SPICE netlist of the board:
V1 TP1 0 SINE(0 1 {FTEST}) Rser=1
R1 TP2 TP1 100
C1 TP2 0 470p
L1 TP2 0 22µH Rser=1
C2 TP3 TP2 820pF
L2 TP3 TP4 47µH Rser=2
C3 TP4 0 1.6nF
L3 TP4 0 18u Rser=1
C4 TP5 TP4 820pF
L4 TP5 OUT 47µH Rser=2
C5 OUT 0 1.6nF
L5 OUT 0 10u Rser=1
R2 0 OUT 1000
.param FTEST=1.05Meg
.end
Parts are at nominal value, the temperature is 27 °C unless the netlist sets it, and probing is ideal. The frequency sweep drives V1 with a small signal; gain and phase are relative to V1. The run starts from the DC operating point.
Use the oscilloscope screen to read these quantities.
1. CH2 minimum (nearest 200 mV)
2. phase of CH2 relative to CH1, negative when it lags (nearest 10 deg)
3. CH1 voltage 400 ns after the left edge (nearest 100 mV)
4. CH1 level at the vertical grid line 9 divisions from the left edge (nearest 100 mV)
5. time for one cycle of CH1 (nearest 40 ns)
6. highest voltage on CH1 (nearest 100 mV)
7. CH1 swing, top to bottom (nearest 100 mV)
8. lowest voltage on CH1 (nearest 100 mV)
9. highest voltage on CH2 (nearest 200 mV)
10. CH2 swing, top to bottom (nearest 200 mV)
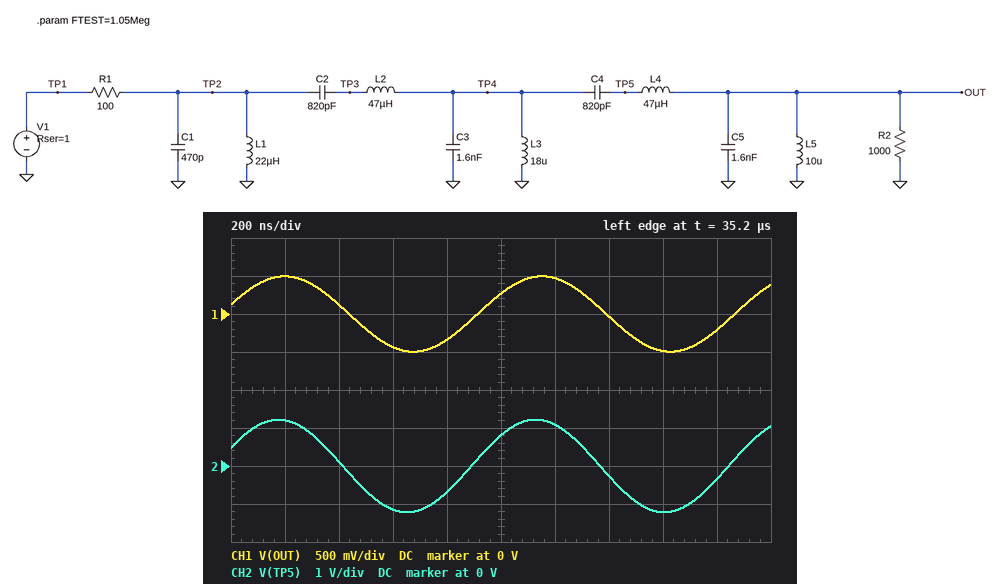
-1.2 V
10 deg
100 mV
-200 mV
960 ns
500 mV
1.0 V
-500 mV
1.2 V
2.4 V
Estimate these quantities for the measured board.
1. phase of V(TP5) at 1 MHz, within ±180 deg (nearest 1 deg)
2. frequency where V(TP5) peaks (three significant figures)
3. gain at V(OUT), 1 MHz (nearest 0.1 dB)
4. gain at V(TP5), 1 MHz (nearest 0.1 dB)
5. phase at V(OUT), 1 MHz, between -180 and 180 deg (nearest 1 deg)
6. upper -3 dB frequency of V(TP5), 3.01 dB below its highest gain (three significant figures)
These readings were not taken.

32 deg
713 kHz
-7.8 dB
1.0 dB
25 deg
768 kHz
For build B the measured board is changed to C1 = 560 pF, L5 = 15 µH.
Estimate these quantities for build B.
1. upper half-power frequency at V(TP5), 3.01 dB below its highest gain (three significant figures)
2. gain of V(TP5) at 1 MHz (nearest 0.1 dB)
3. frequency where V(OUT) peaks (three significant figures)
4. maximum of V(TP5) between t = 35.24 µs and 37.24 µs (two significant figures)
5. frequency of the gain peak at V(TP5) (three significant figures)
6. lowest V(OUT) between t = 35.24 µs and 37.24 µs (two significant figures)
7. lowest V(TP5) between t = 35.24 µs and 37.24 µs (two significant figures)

1.52 MHz
0.2 dB
1.11 MHz
1.1 V
1.47 MHz
-1.2 V
-1.1 V
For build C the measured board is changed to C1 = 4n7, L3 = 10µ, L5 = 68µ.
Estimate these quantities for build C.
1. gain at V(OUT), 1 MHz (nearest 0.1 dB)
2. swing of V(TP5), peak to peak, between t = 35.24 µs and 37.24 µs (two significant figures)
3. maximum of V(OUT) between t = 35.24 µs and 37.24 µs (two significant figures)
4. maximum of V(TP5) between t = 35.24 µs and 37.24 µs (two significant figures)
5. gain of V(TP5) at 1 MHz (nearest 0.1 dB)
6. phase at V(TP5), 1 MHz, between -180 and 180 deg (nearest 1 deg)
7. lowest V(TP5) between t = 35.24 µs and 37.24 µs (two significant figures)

0.5 dB
1.4 V
430 mV
690 mV
2.9 dB
-14 deg
-690 mV
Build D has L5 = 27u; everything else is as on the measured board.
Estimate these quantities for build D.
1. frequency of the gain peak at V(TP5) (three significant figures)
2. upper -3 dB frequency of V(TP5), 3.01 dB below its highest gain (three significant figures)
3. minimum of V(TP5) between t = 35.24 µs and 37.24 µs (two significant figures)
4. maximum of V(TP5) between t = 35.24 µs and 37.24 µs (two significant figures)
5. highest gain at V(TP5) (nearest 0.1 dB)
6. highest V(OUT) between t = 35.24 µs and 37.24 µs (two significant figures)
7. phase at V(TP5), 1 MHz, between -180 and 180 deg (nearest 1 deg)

1.43 MHz
1.48 MHz
-640 mV
640 mV
11.8 dB
1.0 V
58 deg
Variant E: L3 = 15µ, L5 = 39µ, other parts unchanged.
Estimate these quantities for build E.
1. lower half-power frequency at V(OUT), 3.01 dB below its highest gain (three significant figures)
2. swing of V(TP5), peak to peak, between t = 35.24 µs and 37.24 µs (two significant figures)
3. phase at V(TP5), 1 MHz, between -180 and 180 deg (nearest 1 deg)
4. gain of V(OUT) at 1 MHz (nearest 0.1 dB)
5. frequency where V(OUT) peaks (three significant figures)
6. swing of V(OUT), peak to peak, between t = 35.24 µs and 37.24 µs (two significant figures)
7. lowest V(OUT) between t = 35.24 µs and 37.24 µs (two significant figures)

881 kHz
1.7 V
70 deg
0.9 dB
948 kHz
1.5 V
-760 mV
